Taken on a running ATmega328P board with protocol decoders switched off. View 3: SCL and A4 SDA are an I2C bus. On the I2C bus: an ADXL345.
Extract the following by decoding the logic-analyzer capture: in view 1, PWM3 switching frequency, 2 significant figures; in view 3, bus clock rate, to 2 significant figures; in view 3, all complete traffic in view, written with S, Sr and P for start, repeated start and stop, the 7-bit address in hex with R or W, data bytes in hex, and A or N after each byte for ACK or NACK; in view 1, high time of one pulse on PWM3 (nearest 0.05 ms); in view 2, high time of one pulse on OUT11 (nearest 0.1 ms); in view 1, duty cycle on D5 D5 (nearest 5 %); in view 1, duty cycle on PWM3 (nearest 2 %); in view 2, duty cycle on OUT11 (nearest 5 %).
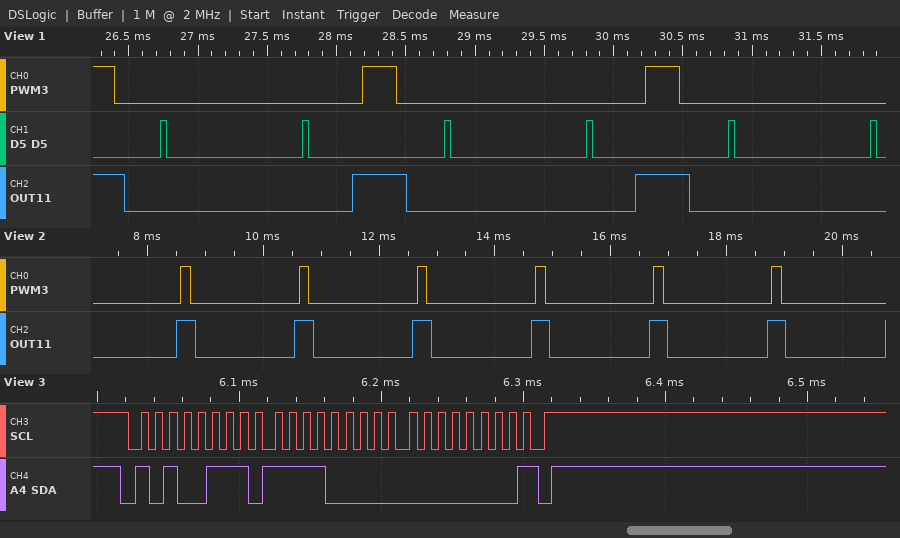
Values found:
490 Hz
100 kHz
S 53R A F0 A 00 N P
0.25 ms
0.3 ms
5 %
12 %
15 %
